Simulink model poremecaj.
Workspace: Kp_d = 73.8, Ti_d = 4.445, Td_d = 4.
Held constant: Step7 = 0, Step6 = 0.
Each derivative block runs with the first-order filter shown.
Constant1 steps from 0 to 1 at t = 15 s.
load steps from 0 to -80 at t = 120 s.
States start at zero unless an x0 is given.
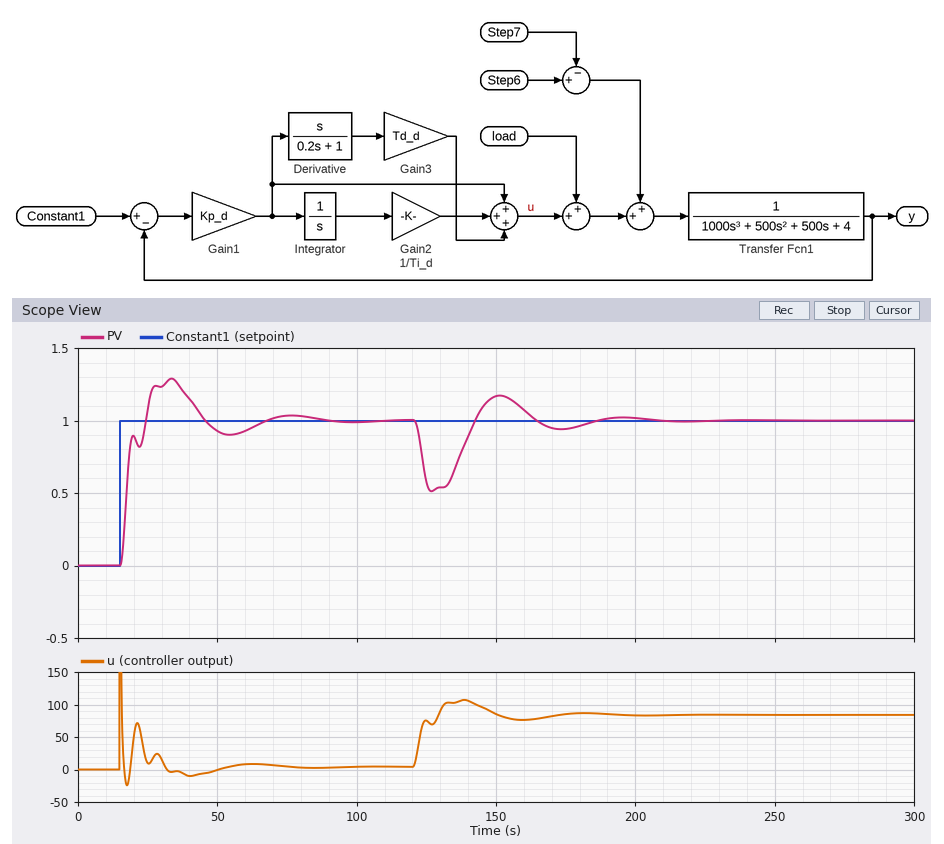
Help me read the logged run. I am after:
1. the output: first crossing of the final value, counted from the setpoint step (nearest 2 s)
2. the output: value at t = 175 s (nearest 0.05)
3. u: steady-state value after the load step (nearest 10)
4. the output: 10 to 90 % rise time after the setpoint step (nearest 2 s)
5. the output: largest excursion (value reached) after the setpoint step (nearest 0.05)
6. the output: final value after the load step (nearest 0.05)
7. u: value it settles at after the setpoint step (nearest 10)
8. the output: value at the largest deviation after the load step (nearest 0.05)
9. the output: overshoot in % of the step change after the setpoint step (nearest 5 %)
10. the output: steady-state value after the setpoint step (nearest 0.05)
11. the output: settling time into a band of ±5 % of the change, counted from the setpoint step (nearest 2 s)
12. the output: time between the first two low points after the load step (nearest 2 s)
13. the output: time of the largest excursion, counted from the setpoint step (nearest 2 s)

10 s
0.95
80
8 s
1.30
1.00
0
0.50
30 %
1.00
48 s
46 s
18 s
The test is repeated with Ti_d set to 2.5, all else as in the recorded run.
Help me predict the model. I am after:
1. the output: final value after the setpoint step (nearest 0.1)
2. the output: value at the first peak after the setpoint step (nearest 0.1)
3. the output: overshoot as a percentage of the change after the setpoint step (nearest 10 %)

1.0
1.4
40 %
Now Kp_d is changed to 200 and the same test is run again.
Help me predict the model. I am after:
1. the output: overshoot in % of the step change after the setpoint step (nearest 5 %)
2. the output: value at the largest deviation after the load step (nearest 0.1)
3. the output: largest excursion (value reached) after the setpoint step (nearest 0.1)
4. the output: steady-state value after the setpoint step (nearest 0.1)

40 %
0.8
1.4
1.0
